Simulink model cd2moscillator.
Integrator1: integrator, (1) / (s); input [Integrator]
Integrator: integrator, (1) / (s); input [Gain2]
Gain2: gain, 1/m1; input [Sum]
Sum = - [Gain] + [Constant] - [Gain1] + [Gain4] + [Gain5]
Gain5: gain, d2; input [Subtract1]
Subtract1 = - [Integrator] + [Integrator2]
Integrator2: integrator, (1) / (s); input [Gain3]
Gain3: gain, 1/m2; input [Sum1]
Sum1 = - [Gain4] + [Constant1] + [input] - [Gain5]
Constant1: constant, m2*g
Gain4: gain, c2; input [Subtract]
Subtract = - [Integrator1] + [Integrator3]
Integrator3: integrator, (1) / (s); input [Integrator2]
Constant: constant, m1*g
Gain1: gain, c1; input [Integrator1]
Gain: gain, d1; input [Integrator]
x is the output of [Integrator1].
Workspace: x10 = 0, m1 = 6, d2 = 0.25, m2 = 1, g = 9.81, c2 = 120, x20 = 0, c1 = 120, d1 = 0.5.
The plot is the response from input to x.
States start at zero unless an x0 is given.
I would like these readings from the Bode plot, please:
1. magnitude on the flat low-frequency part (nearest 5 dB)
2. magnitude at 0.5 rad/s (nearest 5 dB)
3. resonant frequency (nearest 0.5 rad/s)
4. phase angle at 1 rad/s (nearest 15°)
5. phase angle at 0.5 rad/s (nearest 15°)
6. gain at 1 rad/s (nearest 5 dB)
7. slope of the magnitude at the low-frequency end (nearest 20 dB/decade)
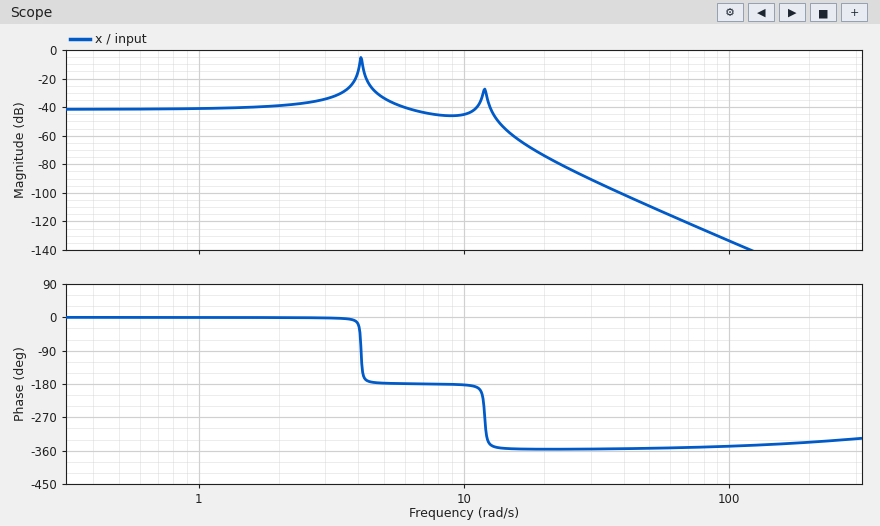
-40 dB
-40 dB
4.0 rad/s
0°
0°
-40 dB
0 dB/decade
